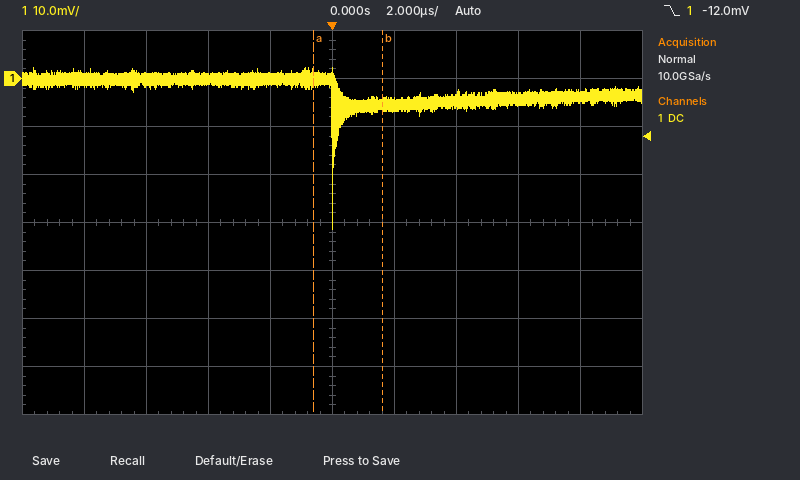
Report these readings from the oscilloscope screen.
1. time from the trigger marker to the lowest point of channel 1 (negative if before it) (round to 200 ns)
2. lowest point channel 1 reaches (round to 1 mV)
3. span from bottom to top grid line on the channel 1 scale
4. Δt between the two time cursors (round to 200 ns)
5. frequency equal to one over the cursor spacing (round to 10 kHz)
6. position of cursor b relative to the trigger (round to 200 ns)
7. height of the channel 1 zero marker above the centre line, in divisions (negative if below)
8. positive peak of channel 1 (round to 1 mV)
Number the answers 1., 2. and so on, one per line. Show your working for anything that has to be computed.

1. 0.0 µs
2. -31 mV
3. 80 mV
4. 2.2 µs
5. 1 / 2.2 µs ≈ 450 kHz
6. +1.6 µs
7. +3.0 div
8. 2 mV
